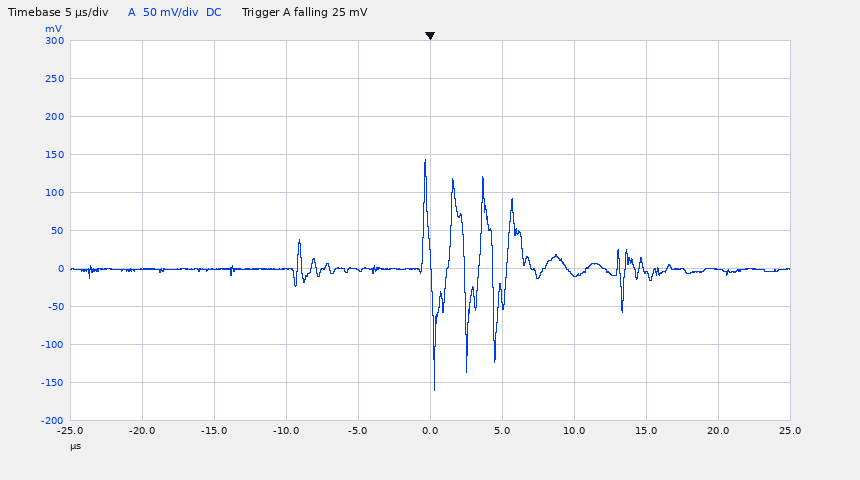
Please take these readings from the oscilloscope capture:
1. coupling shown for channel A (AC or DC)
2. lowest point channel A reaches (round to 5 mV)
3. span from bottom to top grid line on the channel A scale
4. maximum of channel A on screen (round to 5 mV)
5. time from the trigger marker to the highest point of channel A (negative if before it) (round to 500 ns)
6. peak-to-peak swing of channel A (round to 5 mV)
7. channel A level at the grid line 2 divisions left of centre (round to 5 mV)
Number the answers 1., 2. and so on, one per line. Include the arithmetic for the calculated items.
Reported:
1. DC
2. -160 mV
3. 500 mV
4. 145 mV
5. -500 ns
6. 145 mV − (-160 mV) = 305 mV
7. 0 mV
